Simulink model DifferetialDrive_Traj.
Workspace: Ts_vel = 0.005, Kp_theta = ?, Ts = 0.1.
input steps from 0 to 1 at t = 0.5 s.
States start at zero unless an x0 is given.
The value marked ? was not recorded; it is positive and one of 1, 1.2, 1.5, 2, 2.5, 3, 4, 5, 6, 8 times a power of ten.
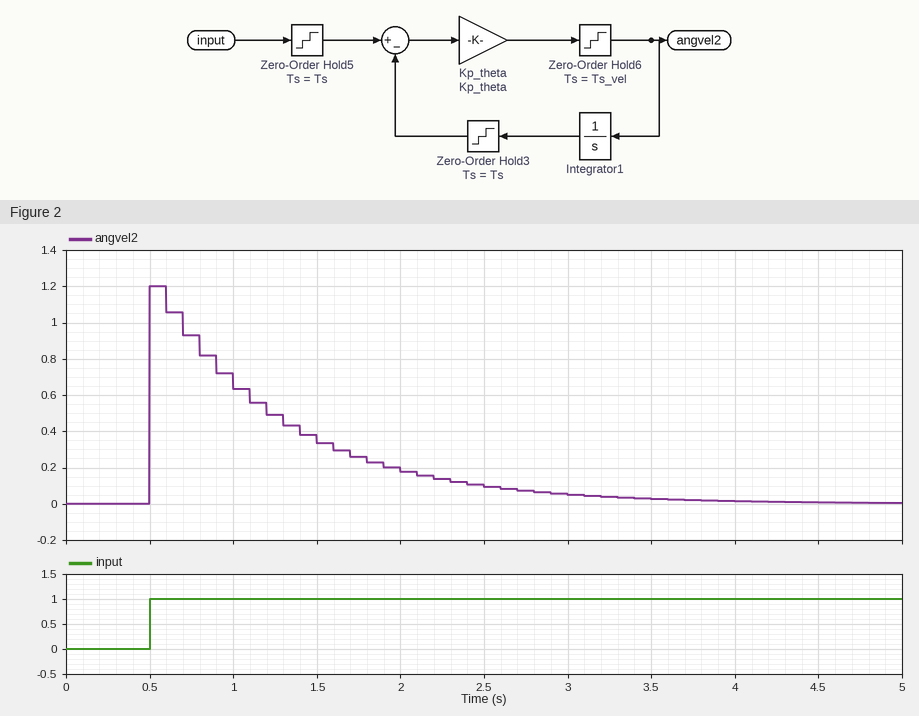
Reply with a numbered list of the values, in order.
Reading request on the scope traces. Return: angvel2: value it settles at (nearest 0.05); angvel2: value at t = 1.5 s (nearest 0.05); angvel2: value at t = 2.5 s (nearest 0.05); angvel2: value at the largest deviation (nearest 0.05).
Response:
1. 0.00
2. 0.35
3. 0.10
4. 1.20
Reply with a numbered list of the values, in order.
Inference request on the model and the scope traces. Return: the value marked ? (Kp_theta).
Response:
1. 1.2
